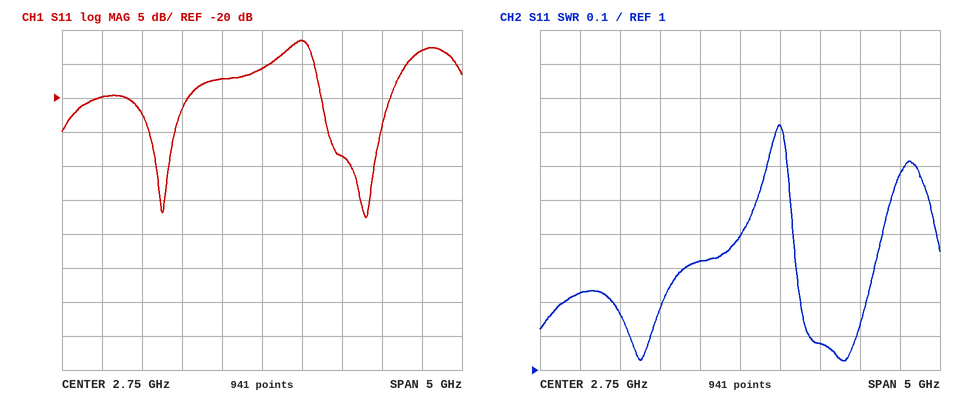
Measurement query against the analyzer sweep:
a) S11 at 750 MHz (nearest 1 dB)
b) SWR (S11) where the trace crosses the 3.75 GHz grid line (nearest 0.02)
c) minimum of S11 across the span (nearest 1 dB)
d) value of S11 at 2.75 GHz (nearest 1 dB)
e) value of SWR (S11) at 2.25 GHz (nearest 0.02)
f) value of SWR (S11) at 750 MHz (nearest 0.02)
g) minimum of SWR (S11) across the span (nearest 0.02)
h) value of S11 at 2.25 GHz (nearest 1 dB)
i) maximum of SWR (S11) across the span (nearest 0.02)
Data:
-20 dB
1.08
-38 dB
-16 dB
1.32
1.22
1.02
-17 dB
1.72
